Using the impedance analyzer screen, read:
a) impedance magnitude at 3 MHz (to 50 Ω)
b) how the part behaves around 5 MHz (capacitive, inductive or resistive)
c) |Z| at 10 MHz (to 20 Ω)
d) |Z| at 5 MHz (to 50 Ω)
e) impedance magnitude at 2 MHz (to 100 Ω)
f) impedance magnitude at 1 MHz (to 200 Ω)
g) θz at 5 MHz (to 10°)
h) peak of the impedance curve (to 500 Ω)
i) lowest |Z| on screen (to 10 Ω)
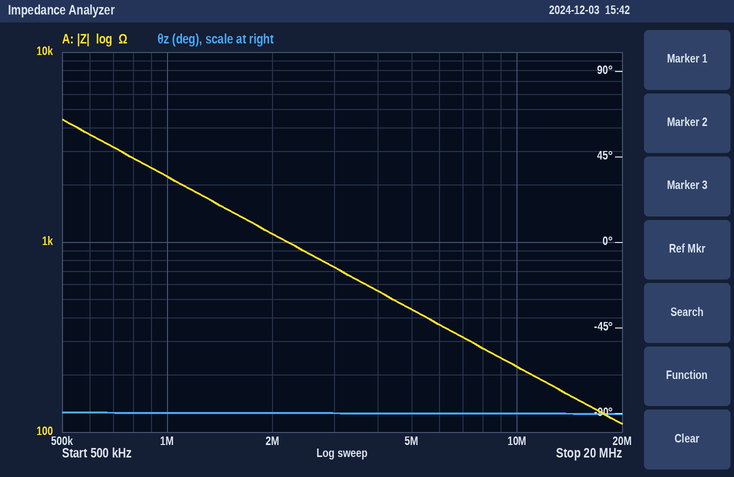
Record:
750 Ω
capacitive
220 Ω
450 Ω
1.1 kΩ
2.2 kΩ
-90°
4.5 kΩ
110 Ω
